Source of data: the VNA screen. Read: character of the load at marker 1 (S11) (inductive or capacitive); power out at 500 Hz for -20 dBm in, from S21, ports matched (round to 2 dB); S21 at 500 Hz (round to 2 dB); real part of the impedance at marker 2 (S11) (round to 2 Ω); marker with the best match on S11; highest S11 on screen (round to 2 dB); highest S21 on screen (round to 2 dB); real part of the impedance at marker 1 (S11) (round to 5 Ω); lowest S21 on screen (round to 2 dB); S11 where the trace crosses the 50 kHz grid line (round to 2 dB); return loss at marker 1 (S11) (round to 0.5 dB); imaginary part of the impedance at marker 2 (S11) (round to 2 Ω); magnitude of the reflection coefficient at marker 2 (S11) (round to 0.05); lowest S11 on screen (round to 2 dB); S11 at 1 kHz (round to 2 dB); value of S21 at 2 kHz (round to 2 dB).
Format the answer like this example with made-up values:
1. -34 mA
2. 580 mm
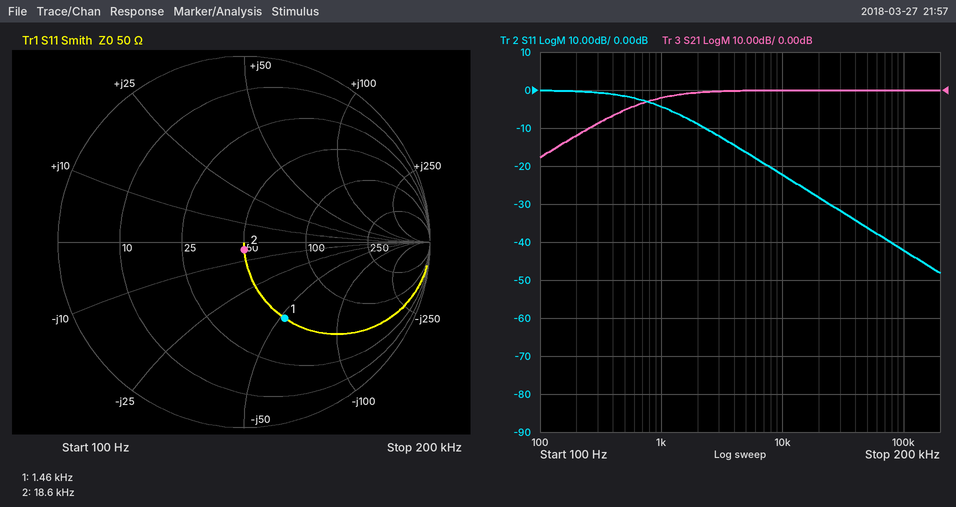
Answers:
1. capacitive
2. -26 dBm
3. -6 dB
4. 50 Ω
5. marker 2
6. 0 dB
7. 0 dB
8. 50 Ω
9. -18 dB
10. -36 dB
11. 6.5 dB
12. -4 Ω
13. 0.05
14. -48 dB
15. -4 dB
16. 0 dB
